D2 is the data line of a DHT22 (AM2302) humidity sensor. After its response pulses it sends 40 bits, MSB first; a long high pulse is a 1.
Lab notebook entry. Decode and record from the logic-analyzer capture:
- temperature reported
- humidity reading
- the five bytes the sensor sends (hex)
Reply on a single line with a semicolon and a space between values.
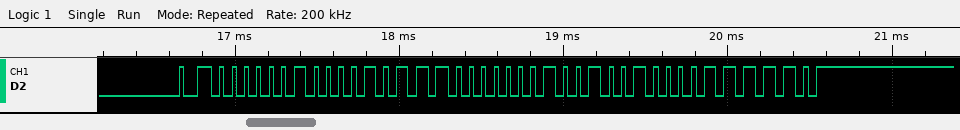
29.2 °C; 53.5 %; 02 17 01 24 3E
